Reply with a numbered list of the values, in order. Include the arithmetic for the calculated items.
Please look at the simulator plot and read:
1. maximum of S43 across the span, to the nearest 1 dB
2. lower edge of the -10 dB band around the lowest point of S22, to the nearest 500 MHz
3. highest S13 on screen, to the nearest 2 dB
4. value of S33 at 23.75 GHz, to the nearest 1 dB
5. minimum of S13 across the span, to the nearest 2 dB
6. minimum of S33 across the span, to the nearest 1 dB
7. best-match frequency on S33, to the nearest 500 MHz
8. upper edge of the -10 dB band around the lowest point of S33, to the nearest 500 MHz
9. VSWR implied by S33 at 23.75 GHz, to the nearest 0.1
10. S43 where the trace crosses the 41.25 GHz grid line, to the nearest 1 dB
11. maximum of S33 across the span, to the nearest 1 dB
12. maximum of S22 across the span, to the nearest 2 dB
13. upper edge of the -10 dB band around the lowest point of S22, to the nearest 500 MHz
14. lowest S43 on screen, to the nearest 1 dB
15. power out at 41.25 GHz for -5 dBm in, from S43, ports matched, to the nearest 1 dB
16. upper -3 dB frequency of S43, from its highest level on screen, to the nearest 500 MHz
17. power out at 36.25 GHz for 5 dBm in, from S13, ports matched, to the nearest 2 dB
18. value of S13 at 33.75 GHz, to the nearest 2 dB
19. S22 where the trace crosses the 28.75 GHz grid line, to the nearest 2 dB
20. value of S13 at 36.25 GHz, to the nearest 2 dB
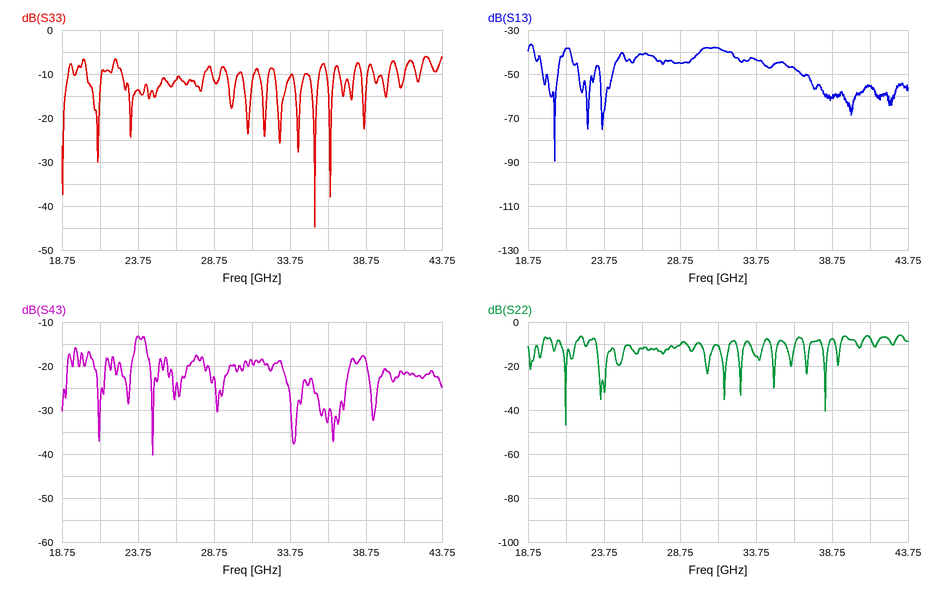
1. -13 dB
2. 21.0 GHz
3. -36 dB
4. -14 dB
5. -90 dB
6. -45 dB
7. 35.5 GHz
8. 35.5 GHz
9. |Γ| = 10^(-14/20) = 0.1995; VSWR = (1 + 0.1995)/(1 − 0.1995) ≈ 1.5
10. -22 dB
11. -6 dB
12. -6 dB
13. 22.0 GHz
14. -40 dB
15. -5 dBm + (-22 dB) = -27 dBm
16. 24.5 GHz
17. 5 dBm + (-48 dB) = -42 dBm
18. -44 dB
19. -10 dB
20. -48 dB
